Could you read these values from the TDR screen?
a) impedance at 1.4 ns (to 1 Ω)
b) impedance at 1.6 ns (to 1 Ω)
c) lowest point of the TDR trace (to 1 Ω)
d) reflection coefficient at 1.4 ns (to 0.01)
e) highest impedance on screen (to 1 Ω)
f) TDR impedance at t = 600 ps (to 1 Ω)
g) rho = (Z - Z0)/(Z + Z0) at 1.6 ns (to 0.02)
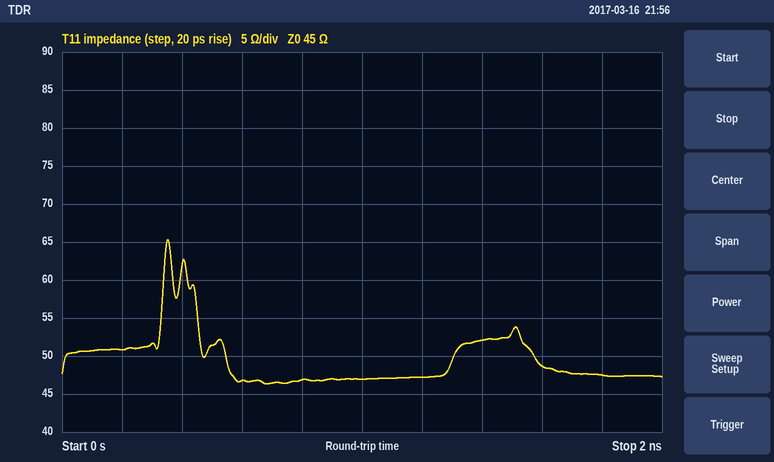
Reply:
52 Ω
49 Ω
46 Ω
+0.07
65 Ω
47 Ω
+0.04
